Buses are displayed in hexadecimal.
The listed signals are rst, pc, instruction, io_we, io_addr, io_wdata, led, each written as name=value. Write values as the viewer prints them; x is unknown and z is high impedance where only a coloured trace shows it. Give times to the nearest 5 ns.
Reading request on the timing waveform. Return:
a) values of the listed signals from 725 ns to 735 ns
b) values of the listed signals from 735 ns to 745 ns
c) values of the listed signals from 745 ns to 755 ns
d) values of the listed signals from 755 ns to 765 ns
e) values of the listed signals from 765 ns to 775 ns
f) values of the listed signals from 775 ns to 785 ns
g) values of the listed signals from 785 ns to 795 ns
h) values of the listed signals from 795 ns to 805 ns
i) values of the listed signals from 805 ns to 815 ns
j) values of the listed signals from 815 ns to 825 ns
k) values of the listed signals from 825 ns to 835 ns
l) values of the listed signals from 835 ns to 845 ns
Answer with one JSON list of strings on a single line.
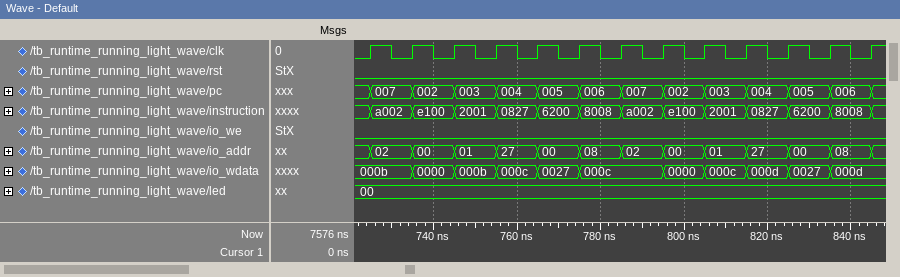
["rst=0, pc=007, instruction=a002, io_we=0, io_addr=02, io_wdata=000b, led=00", "rst=0, pc=002, instruction=e100, io_we=0, io_addr=00, io_wdata=0000, led=00", "rst=0, pc=003, instruction=2001, io_we=0, io_addr=01, io_wdata=000b, led=00", "rst=0, pc=004, instruction=0827, io_we=0, io_addr=27, io_wdata=000c, led=00", "rst=0, pc=005, instruction=6200, io_we=0, io_addr=00, io_wdata=0027, led=00", "rst=0, pc=006, instruction=8008, io_we=0, io_addr=08, io_wdata=000c, led=00", "rst=0, pc=007, instruction=a002, io_we=0, io_addr=02, io_wdata=000c, led=00", "rst=0, pc=002, instruction=e100, io_we=0, io_addr=00, io_wdata=0000, led=00", "rst=0, pc=003, instruction=2001, io_we=0, io_addr=01, io_wdata=000c, led=00", "rst=0, pc=004, instruction=0827, io_we=0, io_addr=27, io_wdata=000d, led=00", "rst=0, pc=005, instruction=6200, io_we=0, io_addr=00, io_wdata=0027, led=00", "rst=0, pc=006, instruction=8008, io_we=0, io_addr=08, io_wdata=000d, led=00"]
